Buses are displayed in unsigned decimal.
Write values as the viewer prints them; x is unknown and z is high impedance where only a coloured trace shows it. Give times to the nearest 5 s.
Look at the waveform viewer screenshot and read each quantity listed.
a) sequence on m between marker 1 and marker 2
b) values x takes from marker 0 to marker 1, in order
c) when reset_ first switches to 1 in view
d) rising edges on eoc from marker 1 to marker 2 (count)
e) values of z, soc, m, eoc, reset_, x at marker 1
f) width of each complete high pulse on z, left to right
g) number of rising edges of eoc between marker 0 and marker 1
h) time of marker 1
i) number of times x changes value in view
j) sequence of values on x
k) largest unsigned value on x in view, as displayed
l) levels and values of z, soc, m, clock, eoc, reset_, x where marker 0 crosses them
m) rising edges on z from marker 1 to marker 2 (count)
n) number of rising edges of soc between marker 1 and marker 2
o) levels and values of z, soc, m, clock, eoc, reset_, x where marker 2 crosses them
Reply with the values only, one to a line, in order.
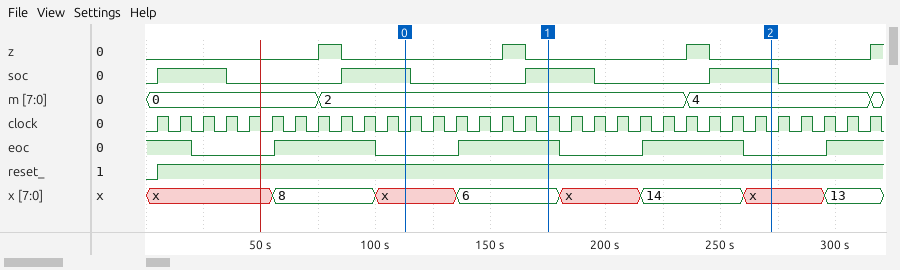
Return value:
2, 4
x, 6
5 s
1
z=0, soc=1, m=2, eoc=1, reset_=1, x=6
10 s, 10 s, 10 s
1
175 s
7
x, 8, x, 6, x, 14, x, 13
14
z=0, soc=1, m=2, clock=0, eoc=0, reset_=1, x=x
1
1
z=0, soc=1, m=4, clock=0, eoc=0, reset_=1, x=x
